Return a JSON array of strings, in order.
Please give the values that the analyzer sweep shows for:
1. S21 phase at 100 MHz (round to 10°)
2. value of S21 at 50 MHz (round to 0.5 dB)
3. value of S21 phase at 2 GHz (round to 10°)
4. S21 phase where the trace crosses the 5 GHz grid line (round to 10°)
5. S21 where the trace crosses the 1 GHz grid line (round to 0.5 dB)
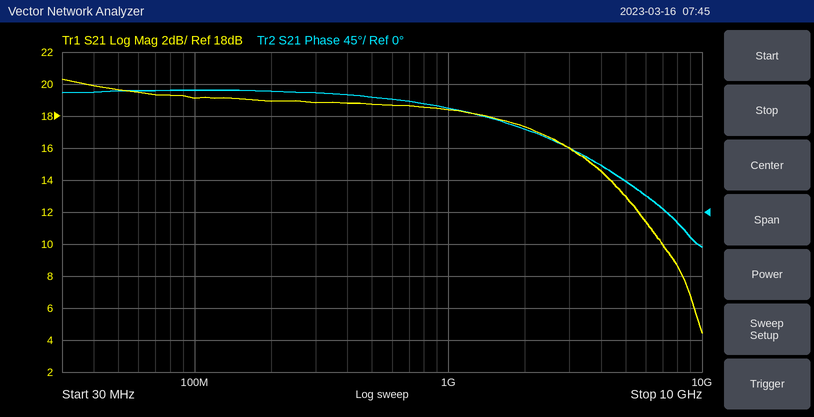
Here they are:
["170°", "19.5 dB", "120°", "40°", "18.5 dB"]
